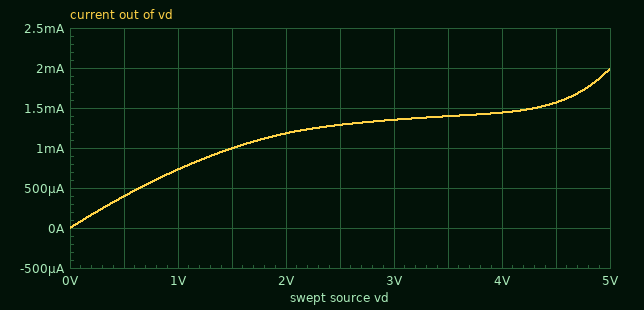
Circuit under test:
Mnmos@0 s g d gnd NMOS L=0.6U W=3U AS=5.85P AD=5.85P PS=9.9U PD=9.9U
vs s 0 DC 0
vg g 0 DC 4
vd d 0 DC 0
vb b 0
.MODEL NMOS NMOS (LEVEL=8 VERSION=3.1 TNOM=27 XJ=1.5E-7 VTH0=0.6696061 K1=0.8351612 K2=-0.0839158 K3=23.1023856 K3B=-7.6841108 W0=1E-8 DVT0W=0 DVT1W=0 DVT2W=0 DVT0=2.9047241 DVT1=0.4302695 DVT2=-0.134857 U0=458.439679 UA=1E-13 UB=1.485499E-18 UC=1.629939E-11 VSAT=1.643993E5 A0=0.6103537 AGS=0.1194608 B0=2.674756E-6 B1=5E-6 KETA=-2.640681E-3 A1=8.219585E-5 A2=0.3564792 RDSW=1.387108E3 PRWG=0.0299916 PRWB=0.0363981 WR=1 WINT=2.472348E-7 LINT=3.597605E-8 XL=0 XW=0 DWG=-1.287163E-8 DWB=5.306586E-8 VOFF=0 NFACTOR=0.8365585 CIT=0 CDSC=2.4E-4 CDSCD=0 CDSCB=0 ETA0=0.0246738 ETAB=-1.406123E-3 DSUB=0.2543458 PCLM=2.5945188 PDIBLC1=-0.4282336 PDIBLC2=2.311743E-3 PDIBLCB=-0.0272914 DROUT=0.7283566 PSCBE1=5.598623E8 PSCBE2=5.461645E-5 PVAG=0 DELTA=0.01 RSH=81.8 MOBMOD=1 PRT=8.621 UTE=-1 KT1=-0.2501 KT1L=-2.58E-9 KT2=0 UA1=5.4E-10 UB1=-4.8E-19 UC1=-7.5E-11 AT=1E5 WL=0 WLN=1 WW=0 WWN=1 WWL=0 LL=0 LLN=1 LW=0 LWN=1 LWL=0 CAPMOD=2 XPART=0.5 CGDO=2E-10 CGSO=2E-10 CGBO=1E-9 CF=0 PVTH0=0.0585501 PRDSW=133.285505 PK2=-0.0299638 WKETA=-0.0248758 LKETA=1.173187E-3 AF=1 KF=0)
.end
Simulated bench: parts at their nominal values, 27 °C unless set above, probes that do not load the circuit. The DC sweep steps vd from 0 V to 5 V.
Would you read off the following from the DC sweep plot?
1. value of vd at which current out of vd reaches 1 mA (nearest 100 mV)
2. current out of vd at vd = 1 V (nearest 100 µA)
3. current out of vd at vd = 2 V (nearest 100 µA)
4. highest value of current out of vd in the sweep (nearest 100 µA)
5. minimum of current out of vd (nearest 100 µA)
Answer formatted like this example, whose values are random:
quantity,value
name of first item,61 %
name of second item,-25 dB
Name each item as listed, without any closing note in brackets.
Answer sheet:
quantity,value
value of vd at which current out of vd reaches 1 mA,1.5 V
current out of vd at vd = 1 V,700 µA
current out of vd at vd = 2 V,1.2 mA
highest value of current out of vd in the sweep,2.0 mA
minimum of current out of vd,0 A
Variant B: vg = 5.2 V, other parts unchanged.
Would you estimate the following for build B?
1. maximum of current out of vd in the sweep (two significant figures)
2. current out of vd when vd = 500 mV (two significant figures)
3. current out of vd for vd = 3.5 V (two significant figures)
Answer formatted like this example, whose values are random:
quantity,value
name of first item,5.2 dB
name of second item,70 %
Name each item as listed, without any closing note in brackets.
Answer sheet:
quantity,value
maximum of current out of vd in the sweep,2.0 mA
current out of vd when vd = 500 mV,410 µA
current out of vd for vd = 3.5 V,1.8 mA
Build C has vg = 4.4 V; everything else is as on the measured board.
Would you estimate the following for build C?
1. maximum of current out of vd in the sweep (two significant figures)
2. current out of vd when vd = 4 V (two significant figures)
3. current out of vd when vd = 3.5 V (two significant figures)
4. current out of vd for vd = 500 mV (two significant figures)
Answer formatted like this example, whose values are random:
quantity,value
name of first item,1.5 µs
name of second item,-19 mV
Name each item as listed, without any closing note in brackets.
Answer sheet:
quantity,value
maximum of current out of vd in the sweep,1.9 mA
current out of vd when vd = 4 V,1.6 mA
current out of vd when vd = 3.5 V,1.5 mA
current out of vd for vd = 500 mV,400 µA
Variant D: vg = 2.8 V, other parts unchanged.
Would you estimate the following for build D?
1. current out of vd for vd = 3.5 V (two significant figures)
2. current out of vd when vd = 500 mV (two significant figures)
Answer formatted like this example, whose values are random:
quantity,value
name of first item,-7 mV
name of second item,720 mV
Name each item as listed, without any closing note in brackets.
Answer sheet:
quantity,value
current out of vd for vd = 3.5 V,910 µA
current out of vd when vd = 500 mV,360 µA
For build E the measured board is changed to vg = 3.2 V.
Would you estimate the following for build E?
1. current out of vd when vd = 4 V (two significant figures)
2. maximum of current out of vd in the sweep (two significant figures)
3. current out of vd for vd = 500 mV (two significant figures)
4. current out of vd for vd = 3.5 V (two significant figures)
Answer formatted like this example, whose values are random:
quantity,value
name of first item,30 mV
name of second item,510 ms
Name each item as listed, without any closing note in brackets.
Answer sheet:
quantity,value
current out of vd when vd = 4 V,1.2 mA
maximum of current out of vd in the sweep,2.3 mA
current out of vd for vd = 500 mV,380 µA
current out of vd for vd = 3.5 V,1.1 mA
